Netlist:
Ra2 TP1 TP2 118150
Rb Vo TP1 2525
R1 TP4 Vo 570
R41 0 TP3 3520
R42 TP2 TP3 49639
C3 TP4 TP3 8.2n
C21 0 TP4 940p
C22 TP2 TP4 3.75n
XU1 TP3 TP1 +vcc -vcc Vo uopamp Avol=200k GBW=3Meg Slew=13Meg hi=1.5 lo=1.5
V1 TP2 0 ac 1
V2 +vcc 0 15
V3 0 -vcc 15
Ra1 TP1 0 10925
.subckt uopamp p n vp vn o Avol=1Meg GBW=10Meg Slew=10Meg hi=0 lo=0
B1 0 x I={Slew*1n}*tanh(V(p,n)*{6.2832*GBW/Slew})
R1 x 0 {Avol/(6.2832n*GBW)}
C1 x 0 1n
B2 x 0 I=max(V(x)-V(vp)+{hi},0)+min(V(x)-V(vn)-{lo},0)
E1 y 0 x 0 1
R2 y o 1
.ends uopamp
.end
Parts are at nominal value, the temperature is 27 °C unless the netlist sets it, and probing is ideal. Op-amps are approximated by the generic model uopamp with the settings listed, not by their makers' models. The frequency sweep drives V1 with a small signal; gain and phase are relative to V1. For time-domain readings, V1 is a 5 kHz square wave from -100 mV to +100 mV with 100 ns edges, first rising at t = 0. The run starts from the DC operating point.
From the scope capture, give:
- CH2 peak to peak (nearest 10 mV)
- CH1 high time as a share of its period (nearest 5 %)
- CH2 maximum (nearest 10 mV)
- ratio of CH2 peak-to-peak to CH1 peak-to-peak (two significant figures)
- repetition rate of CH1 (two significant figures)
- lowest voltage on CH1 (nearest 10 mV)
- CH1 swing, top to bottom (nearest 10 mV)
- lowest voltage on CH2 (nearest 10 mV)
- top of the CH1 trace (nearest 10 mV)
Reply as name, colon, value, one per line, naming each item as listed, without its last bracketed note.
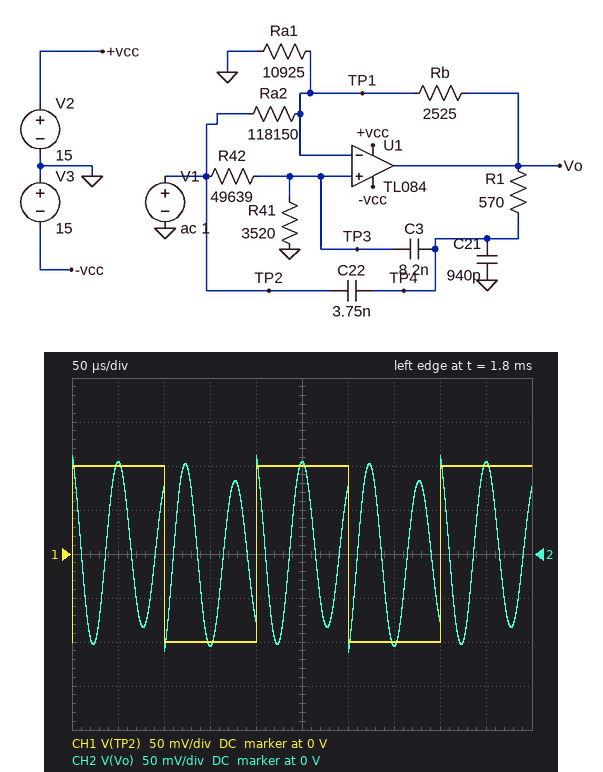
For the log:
CH2 peak to peak: 220 mV
CH1 high time as a share of its period: 50 %
CH2 maximum: 110 mV
ratio of CH2 peak-to-peak to CH1 peak-to-peak: 1.1
repetition rate of CH1: 5.0 kHz
lowest voltage on CH1: -100 mV
CH1 swing, top to bottom: 200 mV
lowest voltage on CH2: -110 mV
top of the CH1 trace: 100 mV
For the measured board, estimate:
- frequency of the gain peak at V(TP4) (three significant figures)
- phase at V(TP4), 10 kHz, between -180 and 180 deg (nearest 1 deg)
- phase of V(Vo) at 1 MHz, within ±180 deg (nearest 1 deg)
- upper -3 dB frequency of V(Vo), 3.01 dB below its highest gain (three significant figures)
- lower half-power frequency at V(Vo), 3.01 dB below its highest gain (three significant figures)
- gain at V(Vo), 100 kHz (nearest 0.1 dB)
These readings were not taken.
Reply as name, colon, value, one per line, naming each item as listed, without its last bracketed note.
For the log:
frequency of the gain peak at V(TP4): 18.5 kHz
phase at V(TP4), 10 kHz, between -180 and 180 deg: 142 deg
phase of V(Vo) at 1 MHz, within ±180 deg: -22 deg
upper -3 dB frequency of V(Vo), 3.01 dB below its highest gain: 19.1 kHz
lower half-power frequency at V(Vo), 3.01 dB below its highest gain: 17.9 kHz
gain at V(Vo), 100 kHz: -0.2 dB
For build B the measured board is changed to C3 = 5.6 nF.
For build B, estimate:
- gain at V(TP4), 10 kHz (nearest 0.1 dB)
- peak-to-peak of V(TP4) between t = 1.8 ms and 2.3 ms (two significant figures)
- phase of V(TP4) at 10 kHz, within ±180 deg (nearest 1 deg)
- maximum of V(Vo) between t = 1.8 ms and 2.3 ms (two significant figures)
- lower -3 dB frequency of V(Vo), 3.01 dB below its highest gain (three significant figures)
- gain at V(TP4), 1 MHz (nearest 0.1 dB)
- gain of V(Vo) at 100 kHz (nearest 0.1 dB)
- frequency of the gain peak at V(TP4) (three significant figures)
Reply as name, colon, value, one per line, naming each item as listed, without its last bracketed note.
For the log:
gain at V(TP4), 10 kHz: -14.3 dB
peak-to-peak of V(TP4) between t = 1.8 ms and 2.3 ms: 270 mV
phase of V(TP4) at 10 kHz, within ±180 deg: 122 deg
maximum of V(Vo) between t = 1.8 ms and 2.3 ms: 170 mV
lower -3 dB frequency of V(Vo), 3.01 dB below its highest gain: 20.8 kHz
gain at V(TP4), 1 MHz: -2.2 dB
gain of V(Vo) at 100 kHz: 0 dB
frequency of the gain peak at V(TP4): 22.5 kHz
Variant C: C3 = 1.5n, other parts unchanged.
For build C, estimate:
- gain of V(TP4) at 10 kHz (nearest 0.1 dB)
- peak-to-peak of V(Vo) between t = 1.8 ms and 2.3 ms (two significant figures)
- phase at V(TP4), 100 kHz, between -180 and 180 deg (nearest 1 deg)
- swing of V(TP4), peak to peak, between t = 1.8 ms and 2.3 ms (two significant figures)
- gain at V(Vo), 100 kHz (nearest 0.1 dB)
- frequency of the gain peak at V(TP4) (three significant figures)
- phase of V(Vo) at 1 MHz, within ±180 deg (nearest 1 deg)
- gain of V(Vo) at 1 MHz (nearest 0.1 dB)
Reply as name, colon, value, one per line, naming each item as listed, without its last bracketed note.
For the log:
gain of V(TP4) at 10 kHz: -17.2 dB
peak-to-peak of V(Vo) between t = 1.8 ms and 2.3 ms: 350 mV
phase at V(TP4), 100 kHz, between -180 and 180 deg: 1 deg
swing of V(TP4), peak to peak, between t = 1.8 ms and 2.3 ms: 300 mV
gain at V(Vo), 100 kHz: 0.8 dB
frequency of the gain peak at V(TP4): 46.6 kHz
phase of V(Vo) at 1 MHz, within ±180 deg: -21 deg
gain of V(Vo) at 1 MHz: -1.1 dB
